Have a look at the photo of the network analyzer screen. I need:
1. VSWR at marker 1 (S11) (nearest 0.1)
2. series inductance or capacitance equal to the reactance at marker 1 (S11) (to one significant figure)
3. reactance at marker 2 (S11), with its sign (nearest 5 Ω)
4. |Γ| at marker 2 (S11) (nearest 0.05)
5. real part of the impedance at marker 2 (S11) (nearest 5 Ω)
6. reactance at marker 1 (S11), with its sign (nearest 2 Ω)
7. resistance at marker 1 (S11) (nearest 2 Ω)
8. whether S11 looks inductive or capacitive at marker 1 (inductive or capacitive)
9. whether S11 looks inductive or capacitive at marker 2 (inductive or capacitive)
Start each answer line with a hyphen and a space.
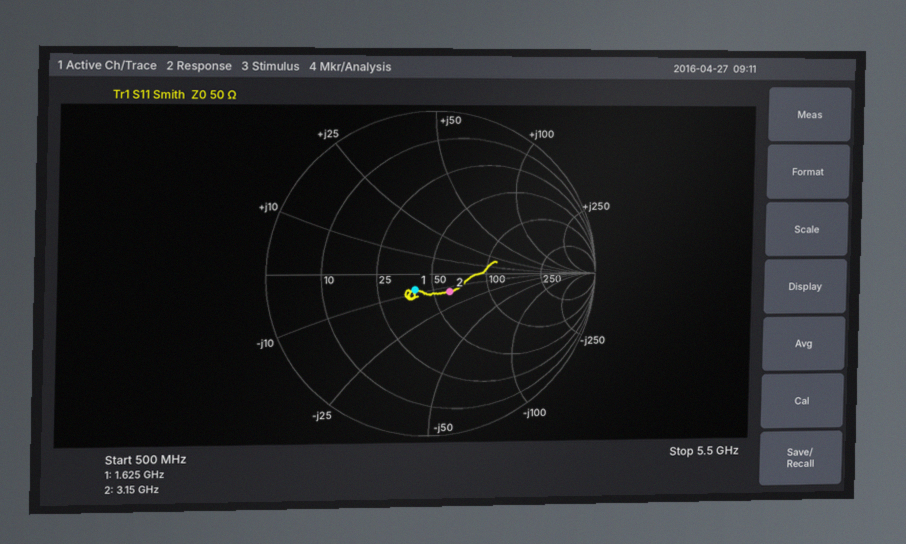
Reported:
- 1.3
- 10 pF
- -15 Ω
- 0.15
- 60 Ω
- -8 Ω
- 40 Ω
- capacitive
- capacitive
